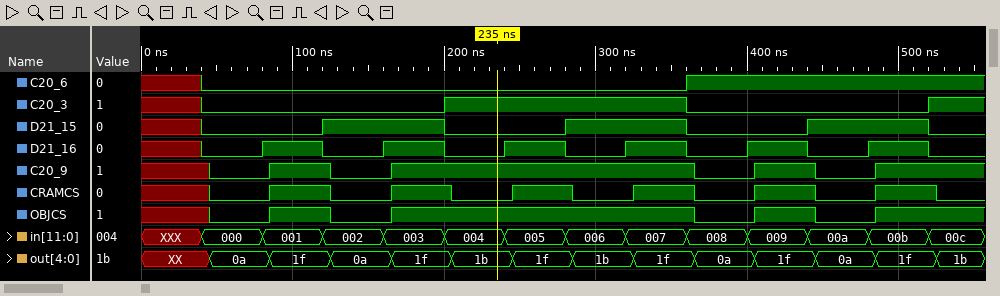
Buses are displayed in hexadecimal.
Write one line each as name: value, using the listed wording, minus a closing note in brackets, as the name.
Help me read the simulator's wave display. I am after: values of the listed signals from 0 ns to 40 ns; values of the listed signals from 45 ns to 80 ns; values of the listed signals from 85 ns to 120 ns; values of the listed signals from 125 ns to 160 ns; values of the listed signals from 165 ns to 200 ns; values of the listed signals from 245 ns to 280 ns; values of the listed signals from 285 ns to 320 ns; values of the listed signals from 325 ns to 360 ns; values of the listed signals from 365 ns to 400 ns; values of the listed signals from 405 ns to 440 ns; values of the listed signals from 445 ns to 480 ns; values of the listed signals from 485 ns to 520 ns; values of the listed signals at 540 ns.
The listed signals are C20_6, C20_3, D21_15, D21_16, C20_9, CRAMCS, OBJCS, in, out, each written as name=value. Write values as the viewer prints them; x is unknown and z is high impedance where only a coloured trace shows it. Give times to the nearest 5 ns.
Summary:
values of the listed signals from 0 ns to 40 ns: C20_6=x, C20_3=x, D21_15=x, D21_16=x, C20_9=x, CRAMCS=x, OBJCS=x, in=XXX, out=XX
values of the listed signals from 45 ns to 80 ns: C20_6=0, C20_3=0, D21_15=0, D21_16=0, C20_9=0, CRAMCS=0, OBJCS=0, in=000, out=0a
values of the listed signals from 85 ns to 120 ns: C20_6=0, C20_3=0, D21_15=0, D21_16=1, C20_9=1, CRAMCS=1, OBJCS=1, in=001, out=1f
values of the listed signals from 125 ns to 160 ns: C20_6=0, C20_3=0, D21_15=1, D21_16=0, C20_9=0, CRAMCS=0, OBJCS=0, in=002, out=0a
values of the listed signals from 165 ns to 200 ns: C20_6=0, C20_3=0, D21_15=1, D21_16=1, C20_9=1, CRAMCS=1, OBJCS=1, in=003, out=1f
values of the listed signals from 245 ns to 280 ns: C20_6=0, C20_3=1, D21_15=0, D21_16=1, C20_9=1, CRAMCS=1, OBJCS=1, in=005, out=1f
values of the listed signals from 285 ns to 320 ns: C20_6=0, C20_3=1, D21_15=1, D21_16=0, C20_9=1, CRAMCS=0, OBJCS=1, in=006, out=1b
values of the listed signals from 325 ns to 360 ns: C20_6=0, C20_3=1, D21_15=1, D21_16=1, C20_9=1, CRAMCS=1, OBJCS=1, in=007, out=1f
values of the listed signals from 365 ns to 400 ns: C20_6=1, C20_3=0, D21_15=0, D21_16=0, C20_9=0, CRAMCS=0, OBJCS=0, in=008, out=0a
values of the listed signals from 405 ns to 440 ns: C20_6=1, C20_3=0, D21_15=0, D21_16=1, C20_9=1, CRAMCS=1, OBJCS=1, in=009, out=1f
values of the listed signals from 445 ns to 480 ns: C20_6=1, C20_3=0, D21_15=1, D21_16=0, C20_9=0, CRAMCS=0, OBJCS=0, in=00a, out=0a
values of the listed signals from 485 ns to 520 ns: C20_6=1, C20_3=0, D21_15=1, D21_16=1, C20_9=1, CRAMCS=1, OBJCS=1, in=00b, out=1f
values of the listed signals at 540 ns: C20_6=1, C20_3=1, D21_15=0, D21_16=0, C20_9=1, CRAMCS=0, OBJCS=1, in=00c, out=1b
